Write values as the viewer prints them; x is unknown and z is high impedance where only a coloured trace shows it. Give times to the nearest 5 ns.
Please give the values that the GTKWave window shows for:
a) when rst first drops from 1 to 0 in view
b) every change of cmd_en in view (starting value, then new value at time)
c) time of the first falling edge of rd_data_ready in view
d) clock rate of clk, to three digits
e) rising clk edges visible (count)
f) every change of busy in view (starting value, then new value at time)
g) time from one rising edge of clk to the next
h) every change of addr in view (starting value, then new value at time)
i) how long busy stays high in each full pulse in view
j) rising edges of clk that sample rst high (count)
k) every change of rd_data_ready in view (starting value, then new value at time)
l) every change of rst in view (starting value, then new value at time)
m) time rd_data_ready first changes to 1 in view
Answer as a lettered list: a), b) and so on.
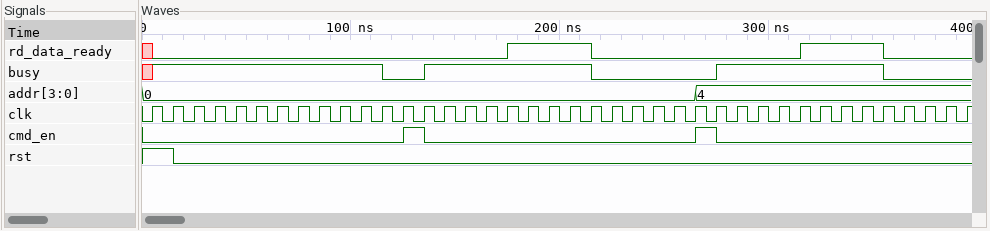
a) 15 ns
b) 0, 1 at 125 ns, 0 at 135 ns, 1 at 265 ns, 0 at 275 ns
c) 215 ns
d) 100 MHz
e) 40
f) x, 1 at 5 ns, 0 at 115 ns, 1 at 135 ns, 0 at 215 ns, 1 at 275 ns, 0 at 355 ns
g) 10 ns
h) 0, 4 at 265 ns
i) 80 ns, 80 ns
j) 2
k) x, 0 at 5 ns, 1 at 175 ns, 0 at 215 ns, 1 at 315 ns, 0 at 355 ns
l) 1, 0 at 15 ns
m) 175 ns
